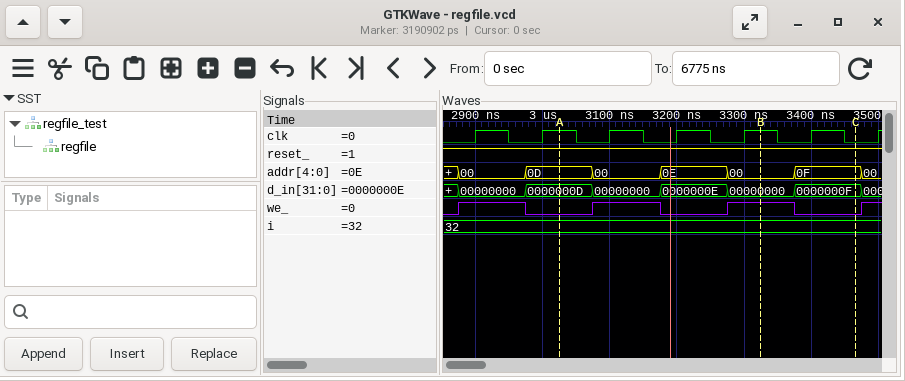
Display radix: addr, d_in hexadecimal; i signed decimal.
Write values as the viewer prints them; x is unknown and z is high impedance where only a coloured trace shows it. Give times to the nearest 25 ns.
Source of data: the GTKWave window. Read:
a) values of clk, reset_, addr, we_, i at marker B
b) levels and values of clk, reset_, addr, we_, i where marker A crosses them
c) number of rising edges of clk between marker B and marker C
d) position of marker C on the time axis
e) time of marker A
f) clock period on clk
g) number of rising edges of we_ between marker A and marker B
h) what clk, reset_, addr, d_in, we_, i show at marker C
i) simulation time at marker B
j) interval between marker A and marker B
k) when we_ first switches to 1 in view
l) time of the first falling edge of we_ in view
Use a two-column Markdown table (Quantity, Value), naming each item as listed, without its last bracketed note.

| Quantity | Value |
|---|---|
| values of clk, reset_, addr, we_, i at marker B | clk=1, reset_=1, addr=00, we_=1, i=32 |
| levels and values of clk, reset_, addr, we_, i where marker A crosses them | clk=1, reset_=1, addr=0D, we_=0, i=32 |
| number of rising edges of clk between marker B and marker C | 1 |
| position of marker C on the time axis | 3475 ns |
| time of marker A | 3025 ns |
| clock period on clk | 100 ns |
| number of rising edges of we_ between marker A and marker B | 2 |
| what clk, reset_, addr, d_in, we_, i show at marker C | clk=0, reset_=1, addr=0F, d_in=0000000F, we_=0, i=32 |
| simulation time at marker B | 3325 ns |
| interval between marker A and marker B | 300 ns |
| when we_ first switches to 1 in view | 2875 ns |
| time of the first falling edge of we_ in view | 2975 ns |
